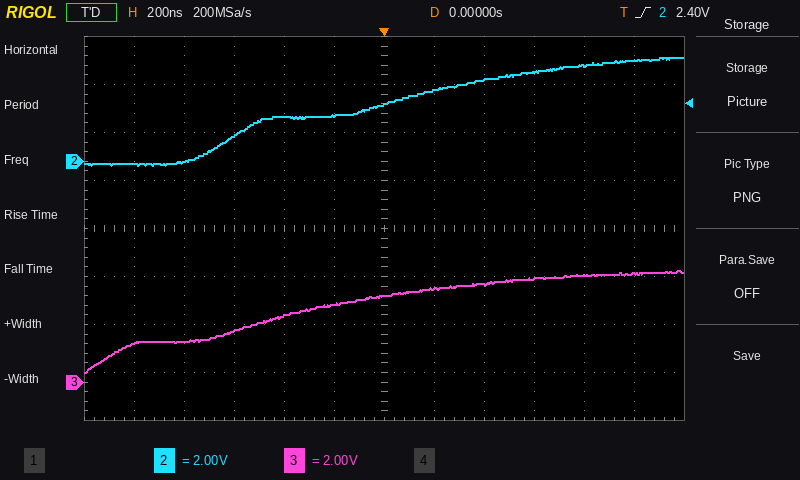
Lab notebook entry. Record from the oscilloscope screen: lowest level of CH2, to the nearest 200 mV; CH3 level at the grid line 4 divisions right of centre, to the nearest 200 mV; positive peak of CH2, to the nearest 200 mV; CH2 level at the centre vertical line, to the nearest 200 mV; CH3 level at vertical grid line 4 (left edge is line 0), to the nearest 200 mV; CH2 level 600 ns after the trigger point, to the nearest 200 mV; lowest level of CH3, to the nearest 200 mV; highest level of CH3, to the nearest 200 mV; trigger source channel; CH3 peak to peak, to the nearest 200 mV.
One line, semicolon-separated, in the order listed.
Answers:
-200 mV; 4.4 V; 4.4 V; 2.4 V; 2.8 V; 3.8 V; 400 mV; 4.6 V; CH2; 4.2 V
